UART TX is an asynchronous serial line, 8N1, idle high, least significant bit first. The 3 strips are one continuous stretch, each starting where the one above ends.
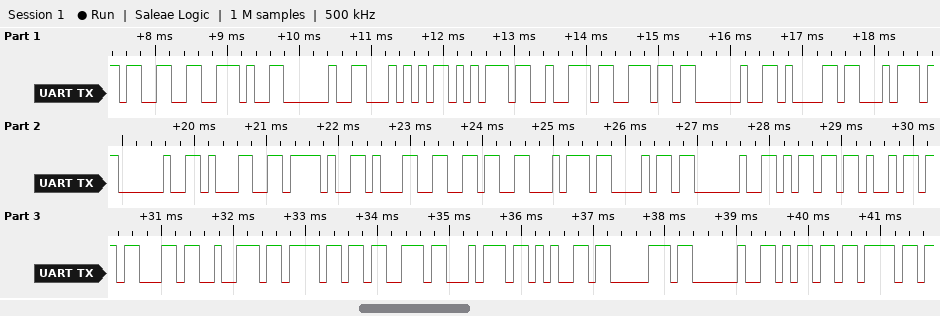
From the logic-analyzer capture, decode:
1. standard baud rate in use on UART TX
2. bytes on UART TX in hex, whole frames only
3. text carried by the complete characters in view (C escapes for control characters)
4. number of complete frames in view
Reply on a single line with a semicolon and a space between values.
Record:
9600 baud; 33 2E 20 54 75 72 6E 20 61 74 20 31 2F 31 36 74 68 20 6D 69 63 72 6F 73 74 65 70 20 6D 6F; "3. Turn at 1/16th microstep mo"; 30
